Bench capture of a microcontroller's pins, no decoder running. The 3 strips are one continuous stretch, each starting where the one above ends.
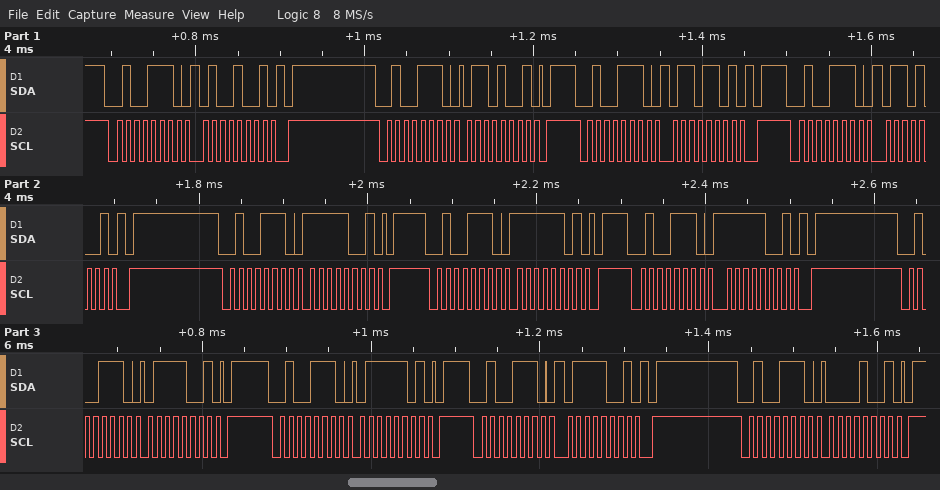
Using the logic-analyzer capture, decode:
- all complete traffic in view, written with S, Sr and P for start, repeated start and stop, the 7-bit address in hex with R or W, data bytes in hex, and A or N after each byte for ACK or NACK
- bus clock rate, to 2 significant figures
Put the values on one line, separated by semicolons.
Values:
S 27W A 49 A P S 27W A 69 A P S 27W A 6D A P S 27W A 69 A P S 27W A F9 A P S 27W A FD A P S 27W A F9 A P S 27W A 79 A P S 27W A 7D A P S 27W A 79 A P S 27W A 09 A P; 100 kHz
